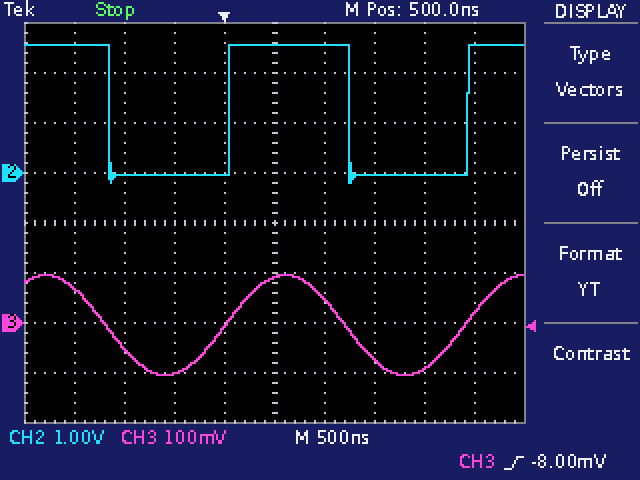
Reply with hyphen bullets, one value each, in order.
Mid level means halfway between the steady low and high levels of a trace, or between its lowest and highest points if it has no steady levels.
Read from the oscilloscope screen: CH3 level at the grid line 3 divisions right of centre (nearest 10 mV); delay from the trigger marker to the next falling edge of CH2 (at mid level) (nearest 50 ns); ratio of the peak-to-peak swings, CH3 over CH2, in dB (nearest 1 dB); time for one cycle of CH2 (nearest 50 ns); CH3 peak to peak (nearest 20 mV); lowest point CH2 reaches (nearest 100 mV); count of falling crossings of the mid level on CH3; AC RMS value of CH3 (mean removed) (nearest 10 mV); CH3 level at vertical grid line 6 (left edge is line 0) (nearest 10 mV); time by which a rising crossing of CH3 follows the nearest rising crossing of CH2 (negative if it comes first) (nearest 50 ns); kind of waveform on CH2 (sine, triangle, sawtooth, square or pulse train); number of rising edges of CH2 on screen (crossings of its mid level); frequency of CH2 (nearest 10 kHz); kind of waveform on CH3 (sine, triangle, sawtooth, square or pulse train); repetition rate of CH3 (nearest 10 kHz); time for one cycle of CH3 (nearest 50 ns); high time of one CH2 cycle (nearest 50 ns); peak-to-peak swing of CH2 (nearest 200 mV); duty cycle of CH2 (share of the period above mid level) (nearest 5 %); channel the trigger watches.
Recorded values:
- -90 mV
- 1.25 µs
- -23 dB
- 2.40 µs
- 200 mV
- -200 mV
- 2
- 70 mV
- 50 mV
- -50 ns
- square
- 2
- 420 kHz
- sine
- 420 kHz
- 2.40 µs
- 1.20 µs
- 2.8 V
- 50 %
- CH3
